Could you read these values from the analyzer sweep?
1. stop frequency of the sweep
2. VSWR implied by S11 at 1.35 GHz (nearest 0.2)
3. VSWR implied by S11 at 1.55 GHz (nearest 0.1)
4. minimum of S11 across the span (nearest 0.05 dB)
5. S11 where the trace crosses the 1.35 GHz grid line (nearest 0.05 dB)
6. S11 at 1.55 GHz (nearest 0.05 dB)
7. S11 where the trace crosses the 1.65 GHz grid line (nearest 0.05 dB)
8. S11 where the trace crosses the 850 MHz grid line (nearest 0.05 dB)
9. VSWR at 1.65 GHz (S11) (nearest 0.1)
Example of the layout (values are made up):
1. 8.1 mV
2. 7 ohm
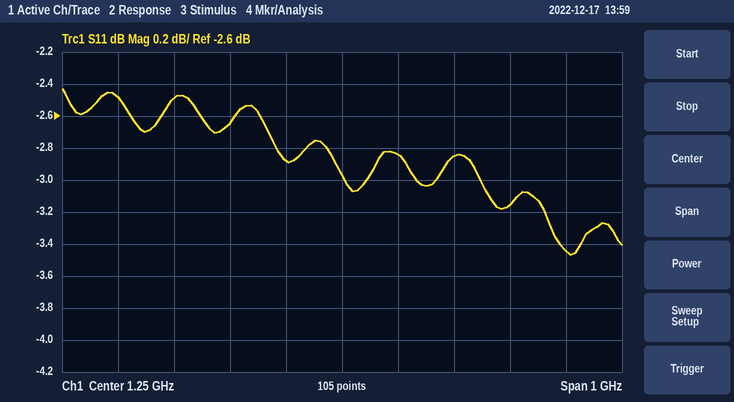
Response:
1. 1.75 GHz
2. 6.2
3. 5.6
4. -3.45 dB
5. -2.85 dB
6. -3.15 dB
7. -3.45 dB
8. -2.50 dB
9. 5.1
